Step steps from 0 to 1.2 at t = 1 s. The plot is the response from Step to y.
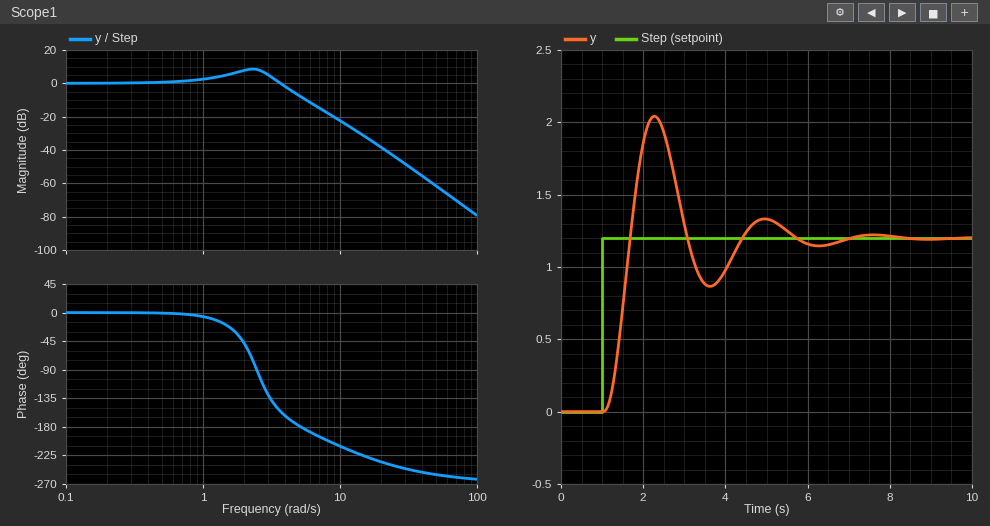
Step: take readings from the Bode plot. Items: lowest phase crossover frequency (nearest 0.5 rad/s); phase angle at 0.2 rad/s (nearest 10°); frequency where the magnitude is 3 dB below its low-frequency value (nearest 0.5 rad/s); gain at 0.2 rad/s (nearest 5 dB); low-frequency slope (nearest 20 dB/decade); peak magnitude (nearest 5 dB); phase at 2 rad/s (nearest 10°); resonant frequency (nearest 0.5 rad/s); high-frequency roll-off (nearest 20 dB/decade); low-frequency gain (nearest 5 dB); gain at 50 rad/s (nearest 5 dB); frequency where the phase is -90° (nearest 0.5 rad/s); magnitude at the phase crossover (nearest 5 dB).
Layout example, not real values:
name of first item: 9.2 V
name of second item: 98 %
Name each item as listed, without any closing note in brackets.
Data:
lowest phase crossover frequency: 5.0 rad/s
phase angle at 0.2 rad/s: 0°
frequency where the magnitude is 3 dB below its low-frequency value: 4.0 rad/s
gain at 0.2 rad/s: 0 dB
low-frequency slope: 0 dB/decade
peak magnitude: 10 dB
phase at 2 rad/s: -50°
resonant frequency: 2.5 rad/s
high-frequency roll-off: -60 dB/decade
low-frequency gain: 0 dB
gain at 50 rad/s: -60 dB
frequency where the phase is -90°: 2.5 rad/s
magnitude at the phase crossover: -10 dB
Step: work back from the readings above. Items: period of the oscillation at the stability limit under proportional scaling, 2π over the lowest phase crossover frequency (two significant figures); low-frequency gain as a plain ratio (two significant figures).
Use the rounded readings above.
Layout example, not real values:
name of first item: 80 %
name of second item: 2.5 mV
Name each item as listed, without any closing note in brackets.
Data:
period of the oscillation at the stability limit under proportional scaling, 2π over the lowest phase crossover frequency: 1.3 s
low-frequency gain as a plain ratio: 1.0
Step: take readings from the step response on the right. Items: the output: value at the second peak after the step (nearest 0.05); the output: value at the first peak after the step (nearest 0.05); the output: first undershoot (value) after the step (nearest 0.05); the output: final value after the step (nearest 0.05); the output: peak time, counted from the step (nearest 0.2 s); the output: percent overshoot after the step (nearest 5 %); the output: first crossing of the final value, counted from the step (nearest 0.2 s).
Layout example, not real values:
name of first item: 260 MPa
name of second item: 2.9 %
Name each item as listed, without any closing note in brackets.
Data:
the output: value at the second peak after the step: 1.35
the output: value at the first peak after the step: 2.05
the output: first undershoot (value) after the step: 0.85
the output: final value after the step: 1.20
the output: peak time, counted from the step: 1.2 s
the output: percent overshoot after the step: 70 %
the output: first crossing of the final value, counted from the step: 0.6 s
